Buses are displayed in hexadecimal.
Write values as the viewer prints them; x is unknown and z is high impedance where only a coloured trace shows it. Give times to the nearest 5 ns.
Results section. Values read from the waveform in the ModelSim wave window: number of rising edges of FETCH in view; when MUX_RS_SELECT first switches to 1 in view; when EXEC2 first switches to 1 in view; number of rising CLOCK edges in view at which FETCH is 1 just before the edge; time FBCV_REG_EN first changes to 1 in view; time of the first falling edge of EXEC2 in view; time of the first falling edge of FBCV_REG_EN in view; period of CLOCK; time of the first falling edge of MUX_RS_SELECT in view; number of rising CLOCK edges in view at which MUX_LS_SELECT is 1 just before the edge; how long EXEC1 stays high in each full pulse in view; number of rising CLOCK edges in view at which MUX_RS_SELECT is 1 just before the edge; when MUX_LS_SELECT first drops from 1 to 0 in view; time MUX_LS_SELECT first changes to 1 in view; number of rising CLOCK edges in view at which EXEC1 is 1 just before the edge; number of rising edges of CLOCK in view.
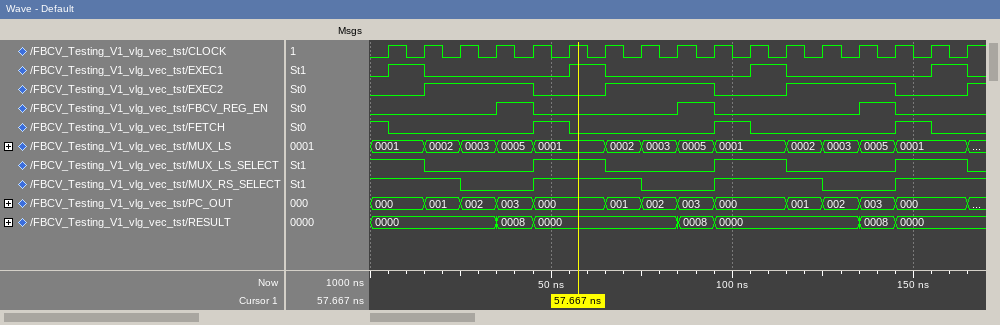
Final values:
3
45 ns
15 ns
4
35 ns
45 ns
45 ns
10 ns
25 ns
8
10 ns, 10 ns, 10 ns, 10 ns
11
15 ns
45 ns
4
17
